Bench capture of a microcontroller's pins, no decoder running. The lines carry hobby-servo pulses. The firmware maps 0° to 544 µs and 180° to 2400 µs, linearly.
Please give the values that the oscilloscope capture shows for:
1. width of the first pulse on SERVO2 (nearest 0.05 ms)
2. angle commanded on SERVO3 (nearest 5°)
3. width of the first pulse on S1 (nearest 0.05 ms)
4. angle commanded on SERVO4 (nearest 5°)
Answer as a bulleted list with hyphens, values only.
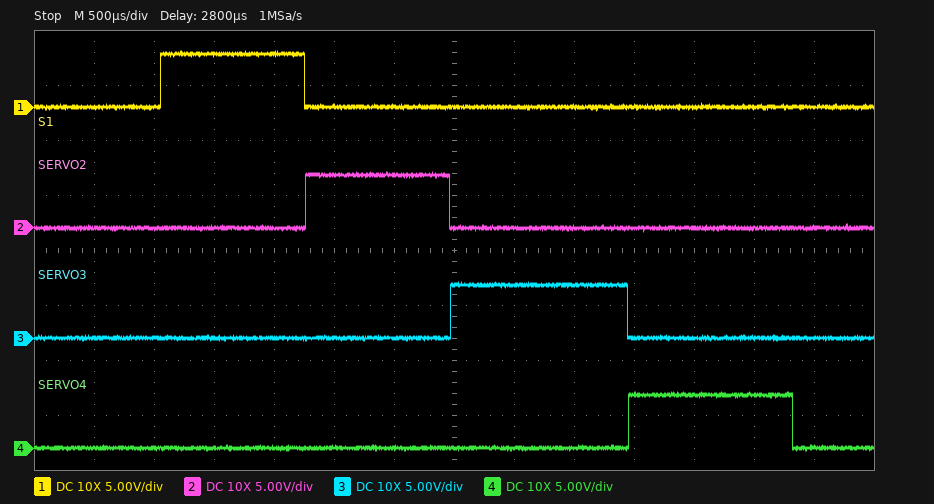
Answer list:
- 1.20 ms
- 90°
- 1.20 ms
- 80°
